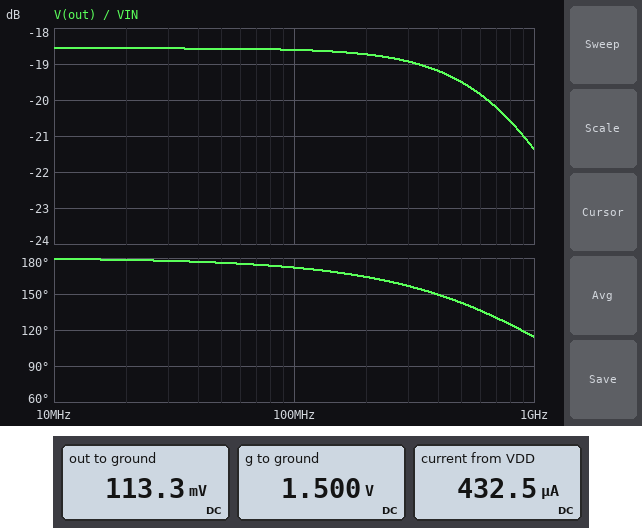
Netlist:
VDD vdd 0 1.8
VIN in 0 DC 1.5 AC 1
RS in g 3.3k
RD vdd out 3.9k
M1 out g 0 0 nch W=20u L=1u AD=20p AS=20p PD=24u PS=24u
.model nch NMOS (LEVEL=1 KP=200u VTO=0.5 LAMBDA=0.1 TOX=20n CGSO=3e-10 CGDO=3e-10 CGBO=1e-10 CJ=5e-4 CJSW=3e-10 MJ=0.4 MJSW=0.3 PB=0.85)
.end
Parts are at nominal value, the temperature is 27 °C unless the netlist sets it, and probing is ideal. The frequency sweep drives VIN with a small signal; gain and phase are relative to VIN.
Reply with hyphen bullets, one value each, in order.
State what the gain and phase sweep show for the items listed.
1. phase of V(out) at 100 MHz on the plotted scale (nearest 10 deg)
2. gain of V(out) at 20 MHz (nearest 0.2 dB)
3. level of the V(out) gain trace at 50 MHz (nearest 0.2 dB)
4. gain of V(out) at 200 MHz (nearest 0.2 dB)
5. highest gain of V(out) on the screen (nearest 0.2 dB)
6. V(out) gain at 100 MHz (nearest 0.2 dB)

- 170 deg
- -18.6 dB
- -18.6 dB
- -18.8 dB
- -18.6 dB
- -18.6 dB
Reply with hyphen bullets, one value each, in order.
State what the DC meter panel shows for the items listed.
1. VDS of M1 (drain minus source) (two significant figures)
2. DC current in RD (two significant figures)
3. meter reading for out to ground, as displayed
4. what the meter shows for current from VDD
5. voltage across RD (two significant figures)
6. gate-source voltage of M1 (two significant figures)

- 110 mV
- 430 µA
- 113.3 mV
- 432.5 µA
- 1.7 V
- 1.5 V
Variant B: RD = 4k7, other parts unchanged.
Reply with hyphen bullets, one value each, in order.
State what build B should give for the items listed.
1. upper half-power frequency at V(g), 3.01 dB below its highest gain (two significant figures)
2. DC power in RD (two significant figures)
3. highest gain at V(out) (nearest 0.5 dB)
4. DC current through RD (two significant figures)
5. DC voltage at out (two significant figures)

- 970 MHz
- 620 µW
- -20.0 dB
- 360 µA
- 94 mV
